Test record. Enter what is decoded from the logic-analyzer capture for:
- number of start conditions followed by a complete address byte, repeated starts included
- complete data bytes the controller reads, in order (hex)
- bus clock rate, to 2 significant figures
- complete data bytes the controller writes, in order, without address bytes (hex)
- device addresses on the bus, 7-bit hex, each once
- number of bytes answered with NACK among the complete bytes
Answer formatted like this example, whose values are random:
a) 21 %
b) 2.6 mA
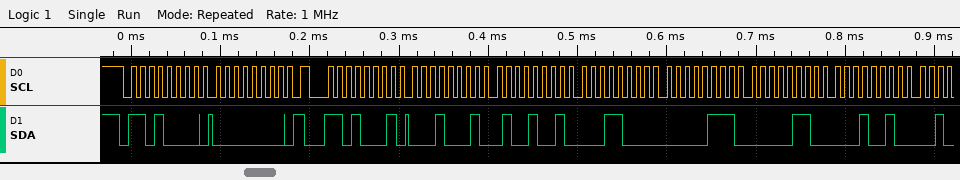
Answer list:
a) 2
b) 11 49 18 07 06 12
c) 100 kHz
d) 00
e) 0x68
f) 0
